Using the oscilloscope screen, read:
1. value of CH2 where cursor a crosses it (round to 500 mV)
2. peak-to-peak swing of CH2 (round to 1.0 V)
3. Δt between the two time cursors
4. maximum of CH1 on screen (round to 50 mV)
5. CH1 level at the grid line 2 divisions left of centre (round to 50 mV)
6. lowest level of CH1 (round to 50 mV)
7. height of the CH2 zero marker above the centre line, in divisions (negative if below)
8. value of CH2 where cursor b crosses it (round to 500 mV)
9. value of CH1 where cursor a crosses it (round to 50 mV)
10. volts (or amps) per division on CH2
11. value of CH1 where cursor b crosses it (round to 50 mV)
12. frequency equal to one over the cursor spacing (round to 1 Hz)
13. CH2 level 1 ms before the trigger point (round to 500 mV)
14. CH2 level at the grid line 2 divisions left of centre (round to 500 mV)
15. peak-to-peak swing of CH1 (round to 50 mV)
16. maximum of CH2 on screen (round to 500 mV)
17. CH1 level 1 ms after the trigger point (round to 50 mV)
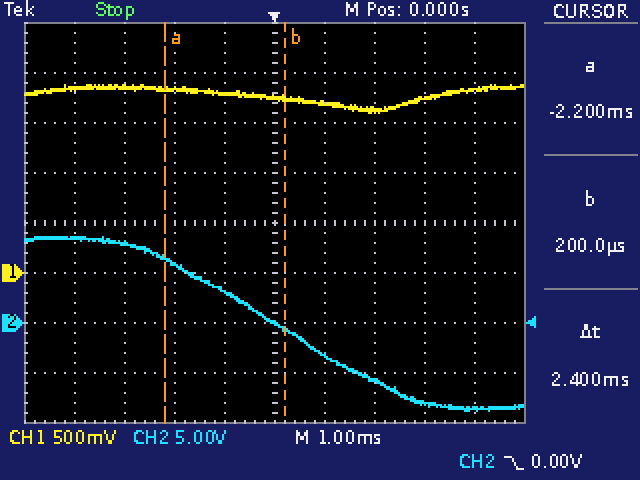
6.5 V
17.0 V
2.4 ms
1.90 V
1.85 V
1.60 V
-2.0 div
-500 mV
1.85 V
5 V
1.75 V
417 Hz
3.0 V
6.0 V
300 mV
8.5 V
1.70 V
